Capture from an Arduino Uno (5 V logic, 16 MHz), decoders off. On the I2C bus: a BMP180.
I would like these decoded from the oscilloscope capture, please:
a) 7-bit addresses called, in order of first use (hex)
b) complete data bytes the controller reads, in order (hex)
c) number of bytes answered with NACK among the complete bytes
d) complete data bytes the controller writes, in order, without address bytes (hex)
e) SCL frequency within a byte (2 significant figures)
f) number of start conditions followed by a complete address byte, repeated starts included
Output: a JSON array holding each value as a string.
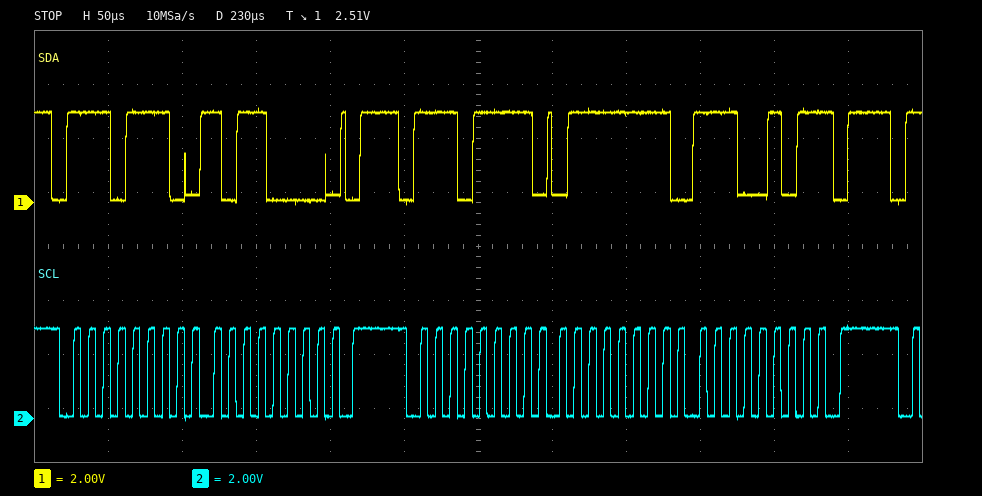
["0x77", "7F E5", "1", "B0", "100 kHz", "2"]
